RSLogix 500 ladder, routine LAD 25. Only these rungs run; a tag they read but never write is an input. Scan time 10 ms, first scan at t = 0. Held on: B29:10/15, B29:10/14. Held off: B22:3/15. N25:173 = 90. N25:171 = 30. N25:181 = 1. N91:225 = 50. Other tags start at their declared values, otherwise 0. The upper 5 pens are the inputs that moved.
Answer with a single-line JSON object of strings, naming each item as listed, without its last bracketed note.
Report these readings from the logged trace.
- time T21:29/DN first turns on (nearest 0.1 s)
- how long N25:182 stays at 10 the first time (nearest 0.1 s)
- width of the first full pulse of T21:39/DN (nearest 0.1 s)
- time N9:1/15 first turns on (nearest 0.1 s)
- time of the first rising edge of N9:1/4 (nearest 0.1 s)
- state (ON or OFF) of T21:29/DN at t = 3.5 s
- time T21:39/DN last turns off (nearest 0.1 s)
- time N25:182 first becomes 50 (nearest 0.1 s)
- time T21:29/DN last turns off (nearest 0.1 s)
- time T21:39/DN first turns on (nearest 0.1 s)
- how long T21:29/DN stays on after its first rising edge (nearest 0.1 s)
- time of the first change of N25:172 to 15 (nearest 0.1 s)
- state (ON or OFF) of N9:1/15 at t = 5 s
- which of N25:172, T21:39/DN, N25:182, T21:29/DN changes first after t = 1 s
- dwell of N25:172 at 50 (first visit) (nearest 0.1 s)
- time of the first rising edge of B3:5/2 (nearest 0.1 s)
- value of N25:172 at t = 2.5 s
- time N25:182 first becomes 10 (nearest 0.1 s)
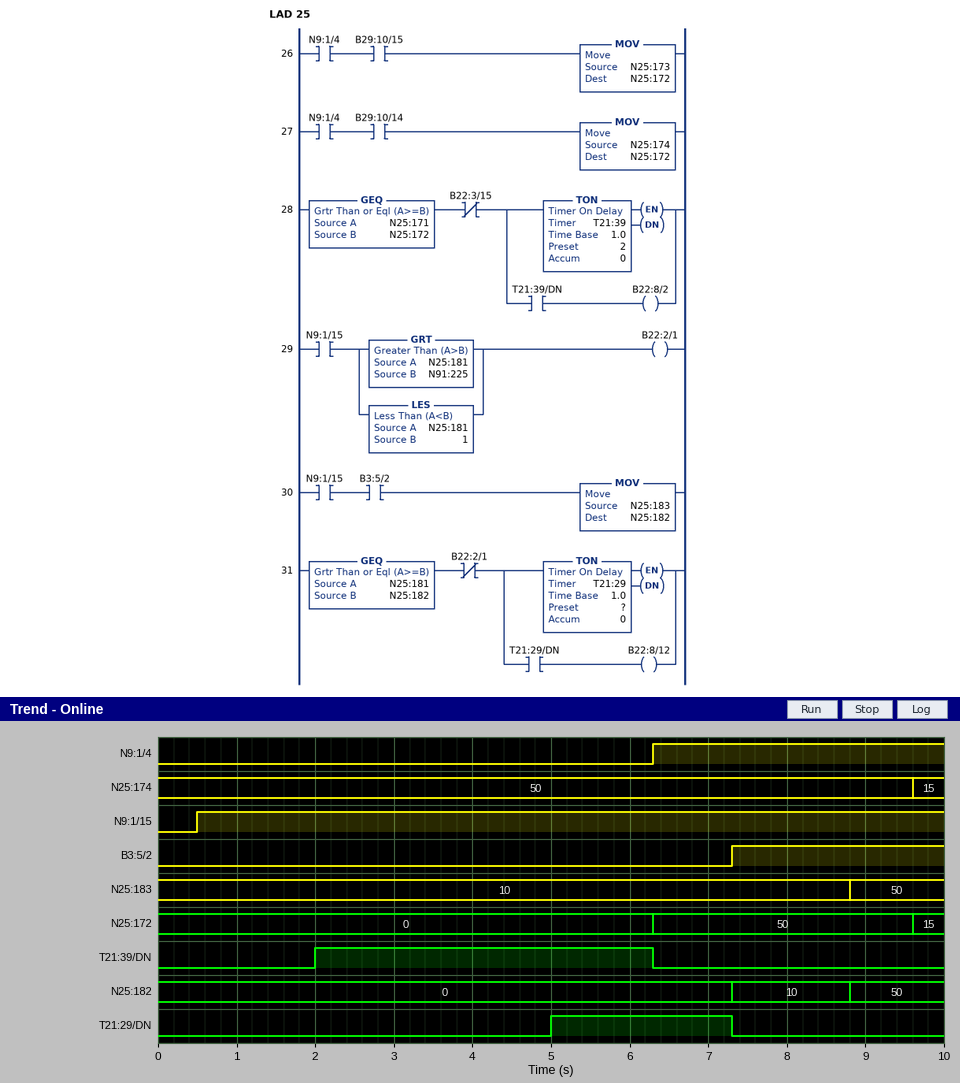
{"time T21:29/DN first turns on": "5.0 s", "how long N25:182 stays at 10 the first time": "1.5 s", "width of the first full pulse of T21:39/DN": "4.3 s", "time N9:1/15 first turns on": "0.5 s", "time of the first rising edge of N9:1/4": "6.3 s", "state (ON or OFF) of T21:29/DN at t = 3.5 s": "OFF", "time T21:39/DN last turns off": "6.3 s", "time N25:182 first becomes 50": "8.8 s", "time T21:29/DN last turns off": "7.3 s", "time T21:39/DN first turns on": "2.0 s", "how long T21:29/DN stays on after its first rising edge": "2.3 s", "time of the first change of N25:172 to 15": "9.6 s", "state (ON or OFF) of N9:1/15 at t = 5 s": "ON", "which of N25:172, T21:39/DN, N25:182, T21:29/DN changes first after t = 1 s": "T21:39/DN", "dwell of N25:172 at 50 (first visit)": "3.3 s", "time of the first rising edge of B3:5/2": "7.3 s", "value of N25:172 at t = 2.5 s": "0", "time N25:182 first becomes 10": "7.3 s"}
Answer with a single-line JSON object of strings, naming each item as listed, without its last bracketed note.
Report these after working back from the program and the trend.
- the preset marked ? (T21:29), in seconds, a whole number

{"the preset marked ? (T21:29), in seconds, a whole number": "5 s"}
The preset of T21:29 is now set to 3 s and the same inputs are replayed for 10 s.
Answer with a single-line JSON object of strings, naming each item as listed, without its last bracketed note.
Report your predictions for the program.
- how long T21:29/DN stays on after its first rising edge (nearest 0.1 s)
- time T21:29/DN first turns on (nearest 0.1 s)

{"how long T21:29/DN stays on after its first rising edge": "4.3 s", "time T21:29/DN first turns on": "3.0 s"}
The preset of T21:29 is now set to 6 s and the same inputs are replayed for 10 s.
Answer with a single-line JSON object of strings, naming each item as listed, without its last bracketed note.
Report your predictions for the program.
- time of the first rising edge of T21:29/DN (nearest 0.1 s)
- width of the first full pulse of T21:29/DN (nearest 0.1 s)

{"time of the first rising edge of T21:29/DN": "6.0 s", "width of the first full pulse of T21:29/DN": "1.3 s"}
